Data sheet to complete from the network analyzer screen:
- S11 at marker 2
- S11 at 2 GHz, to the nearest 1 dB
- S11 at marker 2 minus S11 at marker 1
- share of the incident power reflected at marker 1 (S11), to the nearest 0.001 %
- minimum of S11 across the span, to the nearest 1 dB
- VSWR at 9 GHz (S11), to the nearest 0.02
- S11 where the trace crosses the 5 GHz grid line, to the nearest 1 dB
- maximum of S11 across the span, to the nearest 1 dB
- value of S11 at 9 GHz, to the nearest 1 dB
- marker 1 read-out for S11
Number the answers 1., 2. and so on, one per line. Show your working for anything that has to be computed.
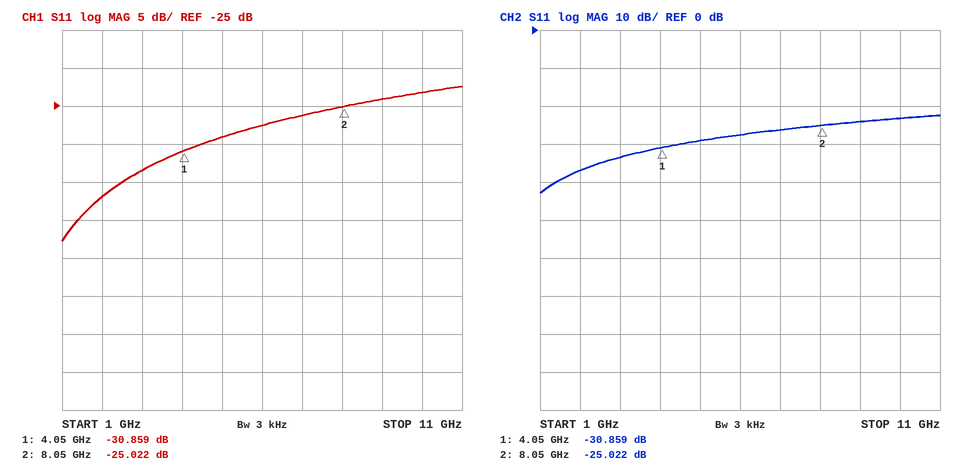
1. -25.022 dB
2. -37 dB
3. -25.022 − (-30.859) = 5.837 dB
4. 10^(-30.859/10) ≈ 0.082 %
5. -43 dB
6. |Γ| = 10^(-24/20) = 0.0631; VSWR = (1 + 0.0631)/(1 − 0.0631) ≈ 1.13, so 1.14 to the nearest 0.02
7. -29 dB
8. -22 dB
9. -24 dB
10. -30.859 dB
